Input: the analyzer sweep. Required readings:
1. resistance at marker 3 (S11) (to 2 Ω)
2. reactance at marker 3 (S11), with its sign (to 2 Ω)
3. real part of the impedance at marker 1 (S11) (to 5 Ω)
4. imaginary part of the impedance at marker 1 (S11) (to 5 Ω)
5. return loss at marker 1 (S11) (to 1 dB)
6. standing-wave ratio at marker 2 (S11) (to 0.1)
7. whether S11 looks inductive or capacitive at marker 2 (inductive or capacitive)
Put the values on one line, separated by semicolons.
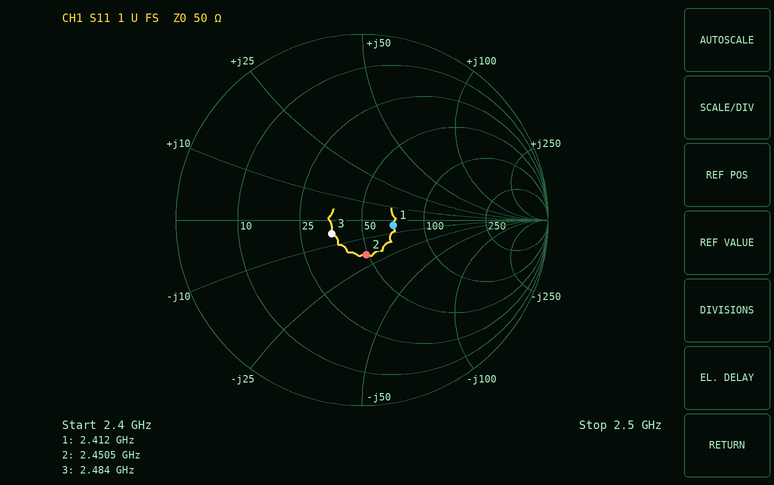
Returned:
36 Ω; -6 Ω; 70 Ω; -5 Ω; 15 dB; 1.5; capacitive
